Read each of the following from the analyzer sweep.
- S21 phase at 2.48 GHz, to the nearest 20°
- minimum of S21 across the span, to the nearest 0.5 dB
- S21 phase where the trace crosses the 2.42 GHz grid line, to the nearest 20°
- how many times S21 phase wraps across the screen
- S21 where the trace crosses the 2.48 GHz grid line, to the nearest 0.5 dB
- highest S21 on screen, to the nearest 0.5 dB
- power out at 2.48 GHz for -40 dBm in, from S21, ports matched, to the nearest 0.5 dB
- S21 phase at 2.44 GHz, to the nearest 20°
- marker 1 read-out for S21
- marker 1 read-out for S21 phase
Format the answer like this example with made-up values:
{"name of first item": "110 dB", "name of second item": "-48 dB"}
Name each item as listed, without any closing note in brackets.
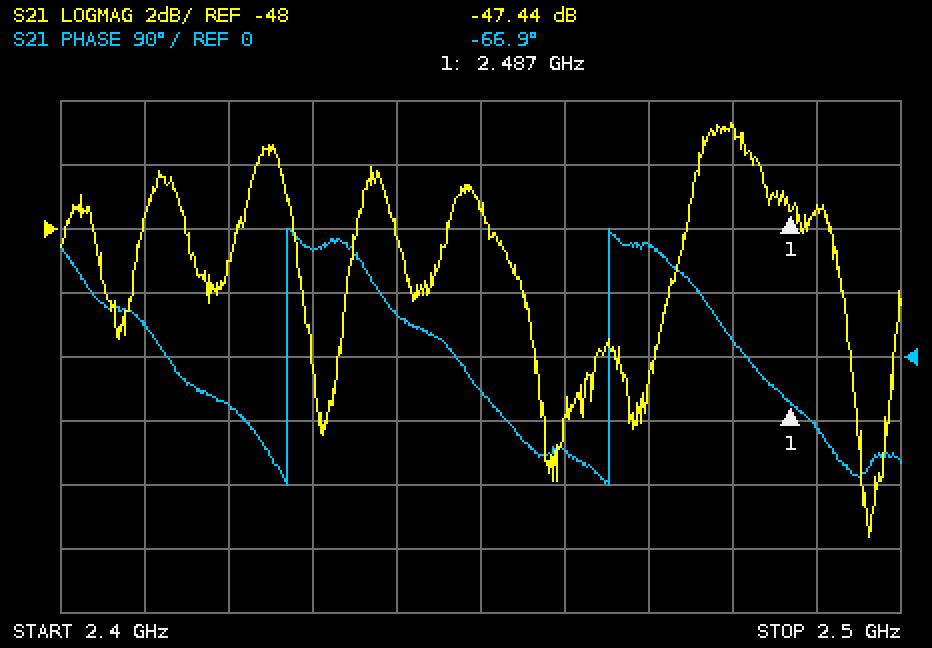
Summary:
{"S21 phase at 2.48 GHz, to the nearest 20°": "20°", "minimum of S21 across the span, to the nearest 0.5 dB": "-57.5 dB", "S21 phase where the trace crosses the 2.42 GHz grid line, to the nearest 20°": "-60°", "how many times S21 phase wraps across the screen": "2", "S21 where the trace crosses the 2.48 GHz grid line, to the nearest 0.5 dB": "-45.0 dB", "highest S21 on screen, to the nearest 0.5 dB": "-44.5 dB", "power out at 2.48 GHz for -40 dBm in, from S21, ports matched, to the nearest 0.5 dB": "-85.0 dBm", "S21 phase at 2.44 GHz, to the nearest 20°": "60°", "marker 1 read-out for S21": "-47.44 dB", "marker 1 read-out for S21 phase": "-66.9°"}
